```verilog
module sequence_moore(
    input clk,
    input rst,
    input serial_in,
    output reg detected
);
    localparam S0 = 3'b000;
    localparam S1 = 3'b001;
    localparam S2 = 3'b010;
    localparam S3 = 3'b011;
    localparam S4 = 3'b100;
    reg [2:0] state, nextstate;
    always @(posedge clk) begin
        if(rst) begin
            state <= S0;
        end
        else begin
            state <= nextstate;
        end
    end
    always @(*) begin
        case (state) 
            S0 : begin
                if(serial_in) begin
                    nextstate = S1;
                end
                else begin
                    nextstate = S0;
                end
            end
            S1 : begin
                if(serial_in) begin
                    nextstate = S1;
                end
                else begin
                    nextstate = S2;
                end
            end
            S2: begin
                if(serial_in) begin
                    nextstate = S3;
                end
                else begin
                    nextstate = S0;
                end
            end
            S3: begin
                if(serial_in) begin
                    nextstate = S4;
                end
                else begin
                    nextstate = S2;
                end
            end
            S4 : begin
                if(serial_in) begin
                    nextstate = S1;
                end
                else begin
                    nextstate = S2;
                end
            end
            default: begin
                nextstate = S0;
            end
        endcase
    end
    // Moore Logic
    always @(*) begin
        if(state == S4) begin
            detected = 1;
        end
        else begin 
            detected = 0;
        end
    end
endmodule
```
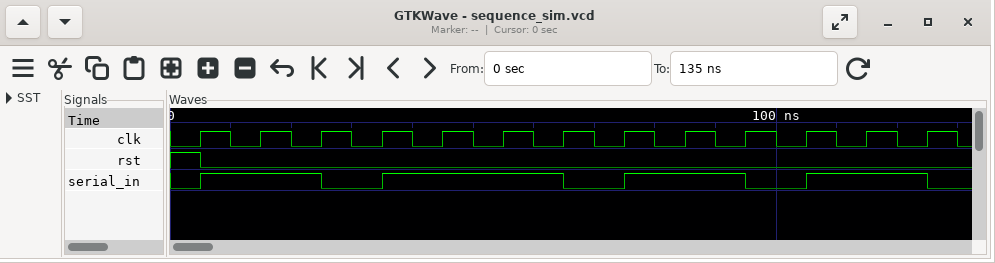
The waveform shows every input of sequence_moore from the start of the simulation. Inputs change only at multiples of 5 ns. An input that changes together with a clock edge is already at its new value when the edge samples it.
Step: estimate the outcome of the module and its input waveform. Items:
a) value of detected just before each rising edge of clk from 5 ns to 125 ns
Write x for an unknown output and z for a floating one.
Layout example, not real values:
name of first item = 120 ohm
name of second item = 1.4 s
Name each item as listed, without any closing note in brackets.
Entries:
value of detected just before each rising edge of clk from 5 ns to 125 ns = x 0 0 0 0 1 0 0 0 1 0 0 1
